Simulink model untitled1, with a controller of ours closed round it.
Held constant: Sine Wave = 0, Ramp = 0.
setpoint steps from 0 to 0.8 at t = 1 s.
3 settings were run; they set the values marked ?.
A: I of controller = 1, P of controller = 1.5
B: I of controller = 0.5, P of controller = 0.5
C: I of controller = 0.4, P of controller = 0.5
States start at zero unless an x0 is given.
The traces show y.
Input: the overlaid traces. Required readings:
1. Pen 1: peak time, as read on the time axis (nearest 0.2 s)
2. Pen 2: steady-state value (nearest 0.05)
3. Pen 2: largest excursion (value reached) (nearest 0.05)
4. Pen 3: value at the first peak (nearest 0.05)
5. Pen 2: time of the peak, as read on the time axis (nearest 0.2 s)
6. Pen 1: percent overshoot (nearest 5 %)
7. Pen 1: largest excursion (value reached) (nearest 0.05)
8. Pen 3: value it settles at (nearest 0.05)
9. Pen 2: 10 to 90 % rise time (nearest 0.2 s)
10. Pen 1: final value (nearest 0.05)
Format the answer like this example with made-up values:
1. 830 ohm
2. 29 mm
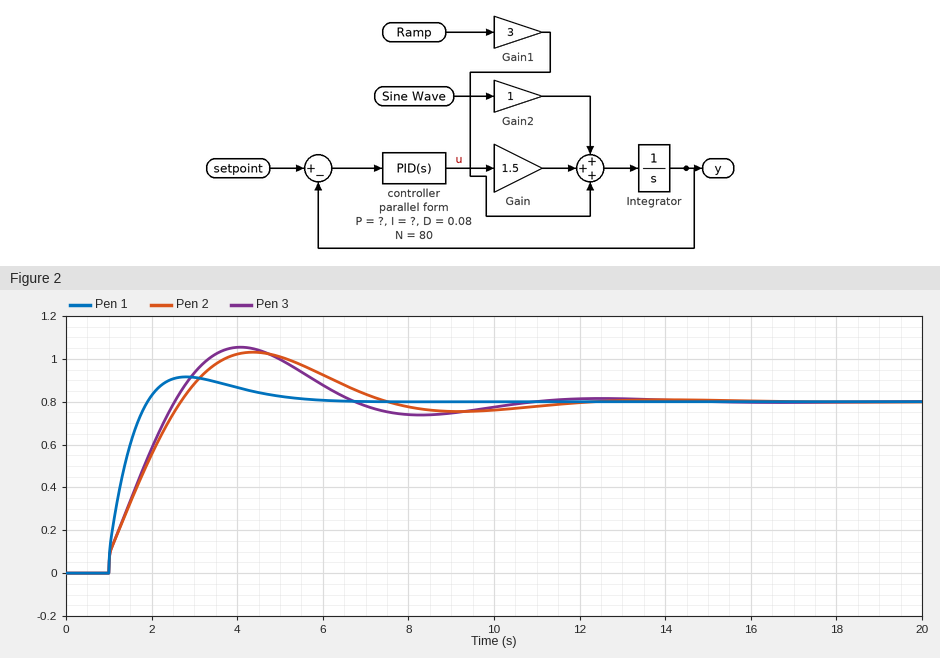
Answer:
1. 2.8 s
2. 0.80
3. 1.05
4. 1.05
5. 4.4 s
6. 15 %
7. 0.90
8. 0.80
9. 1.4 s
10. 0.80
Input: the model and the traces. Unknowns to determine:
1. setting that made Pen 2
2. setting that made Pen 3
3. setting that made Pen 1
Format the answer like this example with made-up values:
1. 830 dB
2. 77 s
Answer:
1. C
2. B
3. A
